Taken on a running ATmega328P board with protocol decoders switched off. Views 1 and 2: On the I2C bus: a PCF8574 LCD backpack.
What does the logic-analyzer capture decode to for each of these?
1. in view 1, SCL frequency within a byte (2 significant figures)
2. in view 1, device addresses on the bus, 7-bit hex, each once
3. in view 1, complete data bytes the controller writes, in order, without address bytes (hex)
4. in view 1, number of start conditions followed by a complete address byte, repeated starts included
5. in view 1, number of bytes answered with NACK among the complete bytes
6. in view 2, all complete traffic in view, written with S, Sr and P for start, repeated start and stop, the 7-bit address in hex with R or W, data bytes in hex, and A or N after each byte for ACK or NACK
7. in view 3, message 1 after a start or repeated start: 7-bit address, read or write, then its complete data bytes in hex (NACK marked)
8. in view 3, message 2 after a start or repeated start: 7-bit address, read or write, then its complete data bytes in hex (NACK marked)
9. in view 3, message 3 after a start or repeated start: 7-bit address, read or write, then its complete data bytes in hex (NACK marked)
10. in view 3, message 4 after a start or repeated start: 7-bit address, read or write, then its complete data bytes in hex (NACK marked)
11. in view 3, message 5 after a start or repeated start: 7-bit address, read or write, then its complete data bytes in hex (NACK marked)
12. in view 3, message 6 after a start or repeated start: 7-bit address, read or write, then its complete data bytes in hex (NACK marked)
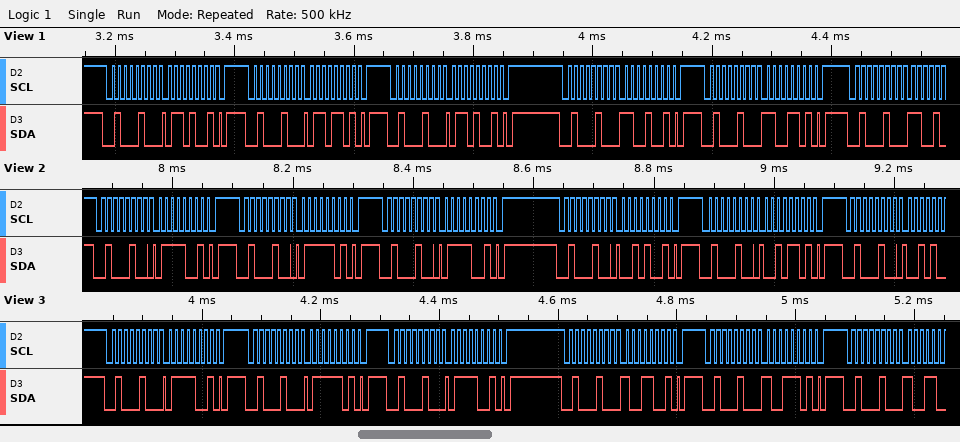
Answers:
100 kHz
0x22
69 6D 69 C9 CD
6
0
S 22W A 79 A P S 22W A 7D A P S 22W A 79 A P S 22W A 29 A P S 22W A 2D A P S 22W A
0x22 write: 79
0x22 write: 7D
0x22 write: 79
0x22 write: 99
0x22 write: 9D
0x22 write
